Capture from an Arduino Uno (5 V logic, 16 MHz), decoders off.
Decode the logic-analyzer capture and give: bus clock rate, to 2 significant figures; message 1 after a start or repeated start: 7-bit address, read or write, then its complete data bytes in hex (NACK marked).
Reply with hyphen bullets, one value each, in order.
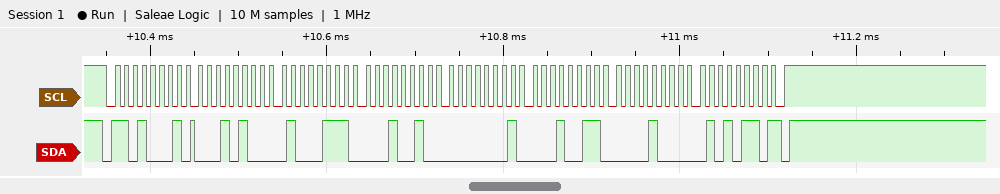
- 100 kHz
- 0x68 read: 14 47 12 01 13 08 56 NACK
